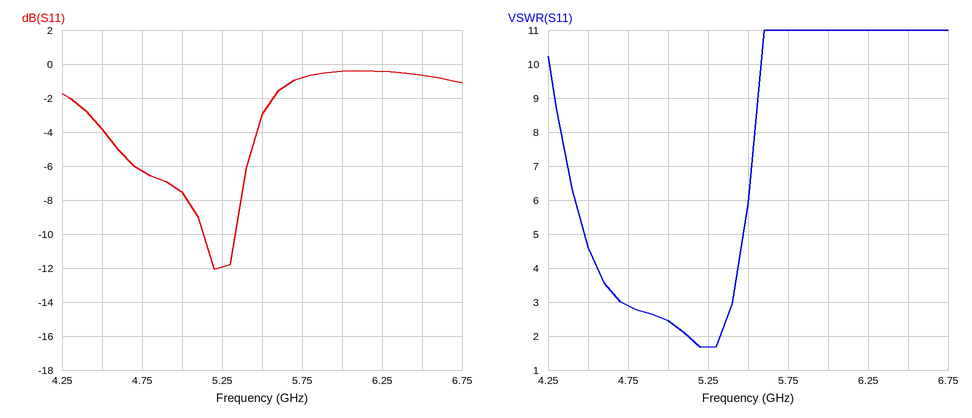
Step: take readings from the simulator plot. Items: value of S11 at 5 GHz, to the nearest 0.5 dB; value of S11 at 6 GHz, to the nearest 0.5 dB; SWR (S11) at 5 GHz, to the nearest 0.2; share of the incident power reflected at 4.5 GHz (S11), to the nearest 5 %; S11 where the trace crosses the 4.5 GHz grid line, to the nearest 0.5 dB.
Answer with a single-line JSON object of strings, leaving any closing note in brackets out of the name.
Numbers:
{"value of S11 at 5 GHz, to the nearest 0.5 dB": "-7.5 dB", "value of S11 at 6 GHz, to the nearest 0.5 dB": "-0.5 dB", "SWR (S11) at 5 GHz, to the nearest 0.2": "2.4", "share of the incident power reflected at 4.5 GHz (S11), to the nearest 5 %": "40 %", "S11 where the trace crosses the 4.5 GHz grid line, to the nearest 0.5 dB": "-4.0 dB"}
